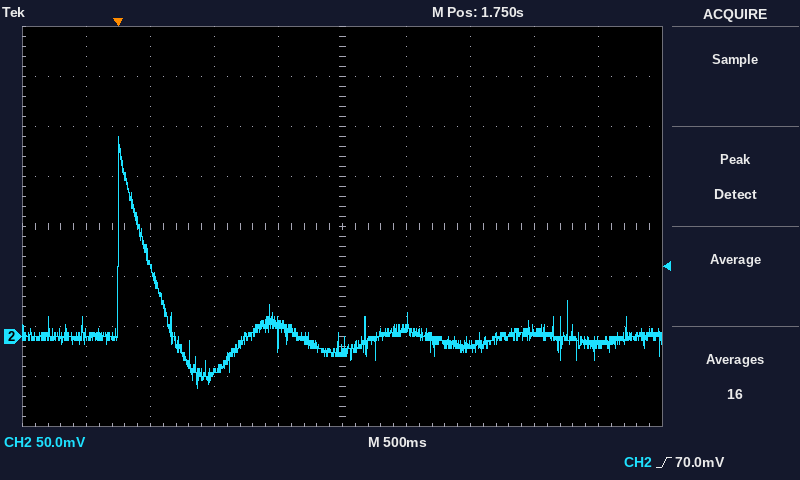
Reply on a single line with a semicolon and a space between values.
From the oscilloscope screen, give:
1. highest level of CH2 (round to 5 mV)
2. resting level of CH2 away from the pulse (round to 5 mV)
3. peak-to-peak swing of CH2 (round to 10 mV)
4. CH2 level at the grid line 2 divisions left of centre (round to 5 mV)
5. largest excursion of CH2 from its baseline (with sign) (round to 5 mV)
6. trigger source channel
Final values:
200 mV; 0 mV; 250 mV; -35 mV; +200 mV; CH2
